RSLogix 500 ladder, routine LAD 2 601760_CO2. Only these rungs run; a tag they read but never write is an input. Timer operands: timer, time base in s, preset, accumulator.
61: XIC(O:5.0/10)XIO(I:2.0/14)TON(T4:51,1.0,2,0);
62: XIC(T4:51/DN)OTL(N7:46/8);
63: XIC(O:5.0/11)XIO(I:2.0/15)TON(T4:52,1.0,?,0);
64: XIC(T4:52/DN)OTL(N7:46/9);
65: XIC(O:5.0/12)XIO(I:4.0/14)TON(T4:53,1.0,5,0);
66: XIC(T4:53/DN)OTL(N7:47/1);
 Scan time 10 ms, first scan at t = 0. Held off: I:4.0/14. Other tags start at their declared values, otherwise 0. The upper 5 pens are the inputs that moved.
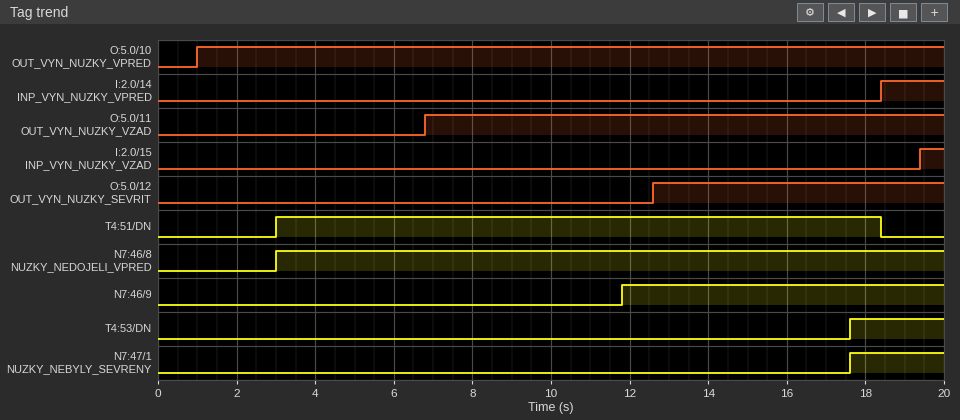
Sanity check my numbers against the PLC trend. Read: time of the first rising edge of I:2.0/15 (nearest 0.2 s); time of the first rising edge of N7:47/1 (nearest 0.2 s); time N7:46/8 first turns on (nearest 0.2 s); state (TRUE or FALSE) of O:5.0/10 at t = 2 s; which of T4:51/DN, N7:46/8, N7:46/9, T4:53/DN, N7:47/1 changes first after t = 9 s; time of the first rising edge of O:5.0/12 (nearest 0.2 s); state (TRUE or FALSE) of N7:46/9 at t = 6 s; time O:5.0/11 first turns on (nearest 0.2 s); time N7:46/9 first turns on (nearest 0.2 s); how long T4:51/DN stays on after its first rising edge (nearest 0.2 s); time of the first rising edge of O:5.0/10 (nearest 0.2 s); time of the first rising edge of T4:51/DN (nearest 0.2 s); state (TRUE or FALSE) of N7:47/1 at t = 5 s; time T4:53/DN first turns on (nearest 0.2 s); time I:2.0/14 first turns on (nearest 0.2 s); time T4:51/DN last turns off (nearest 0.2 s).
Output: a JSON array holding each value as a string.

["19.4 s", "17.6 s", "3.0 s", "TRUE", "N7:46/9", "12.6 s", "FALSE", "6.8 s", "11.8 s", "15.4 s", "1.0 s", "3.0 s", "FALSE", "17.6 s", "18.4 s", "18.4 s"]
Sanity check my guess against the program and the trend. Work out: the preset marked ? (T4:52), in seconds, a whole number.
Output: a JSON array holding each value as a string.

["5 s"]
